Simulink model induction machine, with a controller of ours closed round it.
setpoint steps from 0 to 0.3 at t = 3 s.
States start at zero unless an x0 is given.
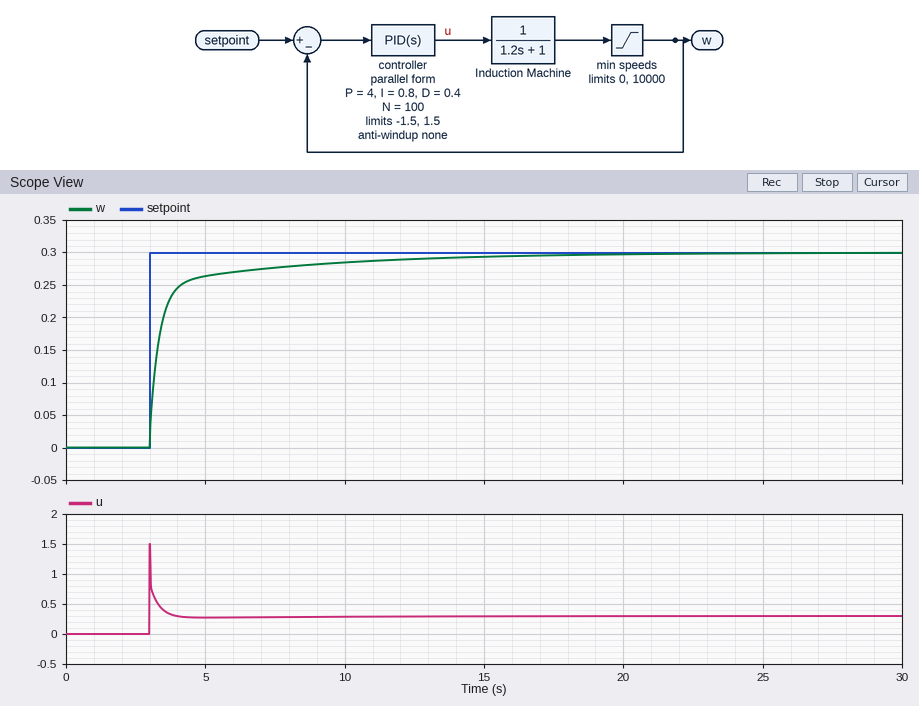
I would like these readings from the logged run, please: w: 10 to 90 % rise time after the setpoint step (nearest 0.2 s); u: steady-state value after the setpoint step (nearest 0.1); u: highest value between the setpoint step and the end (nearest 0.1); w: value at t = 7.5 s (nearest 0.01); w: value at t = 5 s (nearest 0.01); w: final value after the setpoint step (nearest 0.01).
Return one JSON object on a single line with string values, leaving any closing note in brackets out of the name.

{"w: 10 to 90 % rise time after the setpoint step": "3.0 s", "u: steady-state value after the setpoint step": "0.3", "u: highest value between the setpoint step and the end": "1.5", "w: value at t = 7.5 s": "0.28", "w: value at t = 5 s": "0.26", "w: final value after the setpoint step": "0.30"}
